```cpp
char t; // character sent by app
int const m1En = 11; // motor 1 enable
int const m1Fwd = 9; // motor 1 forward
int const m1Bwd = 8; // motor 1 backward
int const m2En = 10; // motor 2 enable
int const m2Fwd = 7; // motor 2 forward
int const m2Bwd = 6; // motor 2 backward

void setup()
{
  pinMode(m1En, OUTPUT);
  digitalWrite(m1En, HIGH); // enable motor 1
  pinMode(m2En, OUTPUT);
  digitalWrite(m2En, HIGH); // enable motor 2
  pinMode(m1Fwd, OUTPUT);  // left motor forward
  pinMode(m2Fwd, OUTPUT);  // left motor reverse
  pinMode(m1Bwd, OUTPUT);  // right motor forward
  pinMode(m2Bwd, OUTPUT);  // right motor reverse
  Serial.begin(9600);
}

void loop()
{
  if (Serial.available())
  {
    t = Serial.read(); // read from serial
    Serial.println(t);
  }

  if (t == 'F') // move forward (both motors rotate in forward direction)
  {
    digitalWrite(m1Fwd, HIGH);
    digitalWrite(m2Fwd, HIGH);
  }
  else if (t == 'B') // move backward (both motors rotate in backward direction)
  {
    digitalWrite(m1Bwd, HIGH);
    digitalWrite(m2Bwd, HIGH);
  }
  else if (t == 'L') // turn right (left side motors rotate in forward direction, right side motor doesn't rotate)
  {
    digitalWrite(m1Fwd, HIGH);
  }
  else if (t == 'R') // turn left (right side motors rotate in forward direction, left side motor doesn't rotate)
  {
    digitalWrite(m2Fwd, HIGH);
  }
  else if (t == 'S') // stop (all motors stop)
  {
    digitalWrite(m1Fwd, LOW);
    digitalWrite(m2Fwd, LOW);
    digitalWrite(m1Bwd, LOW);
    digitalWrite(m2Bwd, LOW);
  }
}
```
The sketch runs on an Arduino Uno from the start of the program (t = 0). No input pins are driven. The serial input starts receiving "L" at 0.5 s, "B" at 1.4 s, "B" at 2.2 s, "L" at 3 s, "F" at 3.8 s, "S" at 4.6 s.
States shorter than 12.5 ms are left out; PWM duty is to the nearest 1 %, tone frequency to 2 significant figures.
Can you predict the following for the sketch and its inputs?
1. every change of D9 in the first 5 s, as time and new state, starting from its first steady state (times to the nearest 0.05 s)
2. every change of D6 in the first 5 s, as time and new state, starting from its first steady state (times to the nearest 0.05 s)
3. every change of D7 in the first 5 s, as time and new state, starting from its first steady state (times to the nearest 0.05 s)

0 s low; 0.5 s high; 4.6 s low
0 s low; 1.4 s high; 4.6 s low
0 s low; 3.8 s high; 4.6 s low
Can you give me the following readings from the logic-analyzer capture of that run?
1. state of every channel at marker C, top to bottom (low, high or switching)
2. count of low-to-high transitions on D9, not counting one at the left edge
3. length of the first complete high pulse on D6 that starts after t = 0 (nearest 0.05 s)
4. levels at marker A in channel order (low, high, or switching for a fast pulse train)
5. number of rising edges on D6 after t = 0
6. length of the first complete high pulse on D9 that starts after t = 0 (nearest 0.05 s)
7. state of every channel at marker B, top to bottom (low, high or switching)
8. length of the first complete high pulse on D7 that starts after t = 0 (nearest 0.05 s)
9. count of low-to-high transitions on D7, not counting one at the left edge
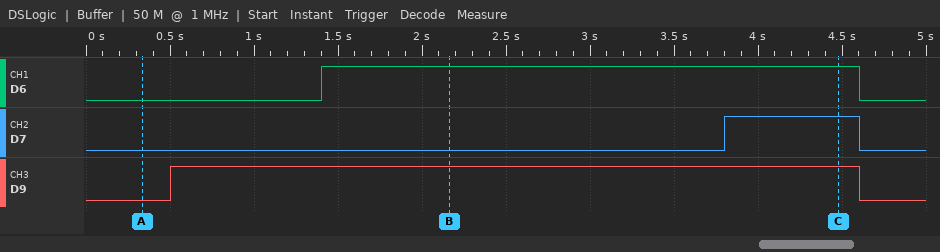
D6 high, D7 high, D9 high
1
3.20 s
D6 low, D7 low, D9 low
1
4.10 s
D6 high, D7 low, D9 high
0.80 s
1
